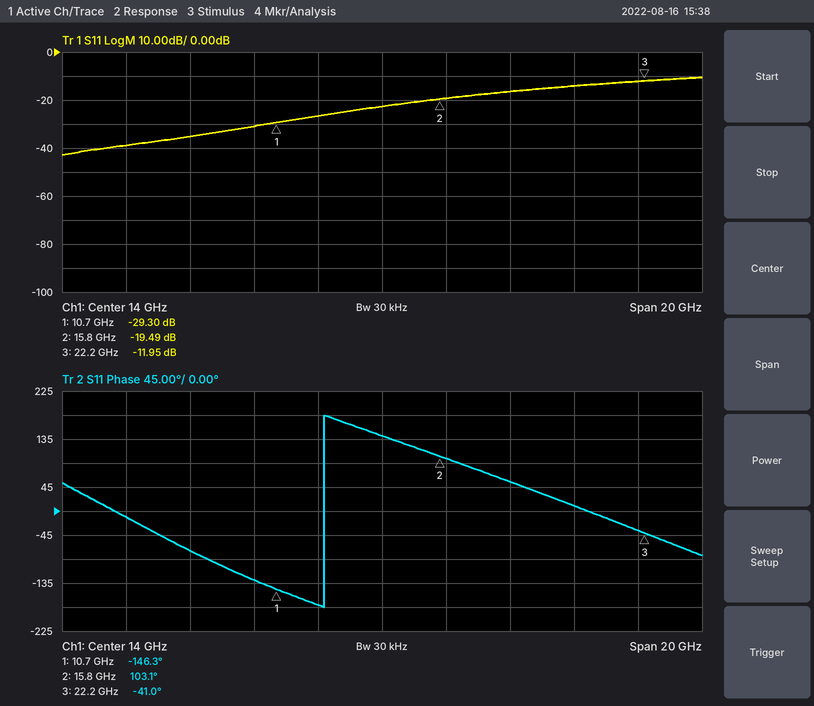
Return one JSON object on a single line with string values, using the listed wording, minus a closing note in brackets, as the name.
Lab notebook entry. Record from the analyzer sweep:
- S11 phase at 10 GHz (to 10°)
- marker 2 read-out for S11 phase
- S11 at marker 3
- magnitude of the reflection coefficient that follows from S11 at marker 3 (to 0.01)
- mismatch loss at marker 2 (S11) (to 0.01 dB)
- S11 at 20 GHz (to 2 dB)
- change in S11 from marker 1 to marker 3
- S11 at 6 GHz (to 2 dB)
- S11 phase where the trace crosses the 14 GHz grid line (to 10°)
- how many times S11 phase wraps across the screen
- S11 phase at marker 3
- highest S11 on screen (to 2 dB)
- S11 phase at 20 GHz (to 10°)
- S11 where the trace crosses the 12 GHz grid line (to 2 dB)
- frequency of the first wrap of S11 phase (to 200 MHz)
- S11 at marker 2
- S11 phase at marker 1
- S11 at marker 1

{"S11 phase at 10 GHz": "-130°", "marker 2 read-out for S11 phase": "103.1°", "S11 at marker 3": "-11.95 dB", "magnitude of the reflection coefficient that follows from S11 at marker 3": "0.25", "mismatch loss at marker 2 (S11)": "0.05 dB", "S11 at 20 GHz": "-14 dB", "change in S11 from marker 1 to marker 3": "17.35 dB", "S11 at 6 GHz": "-38 dB", "S11 phase where the trace crosses the 14 GHz grid line": "140°", "how many times S11 phase wraps across the screen": "1", "S11 phase at marker 3": "-41.0°", "highest S11 on screen": "-10 dB", "S11 phase at 20 GHz": "10°", "S11 where the trace crosses the 12 GHz grid line": "-26 dB", "frequency of the first wrap of S11 phase": "12.2 GHz", "S11 at marker 2": "-19.49 dB", "S11 phase at marker 1": "-146.3°", "S11 at marker 1": "-29.30 dB"}
